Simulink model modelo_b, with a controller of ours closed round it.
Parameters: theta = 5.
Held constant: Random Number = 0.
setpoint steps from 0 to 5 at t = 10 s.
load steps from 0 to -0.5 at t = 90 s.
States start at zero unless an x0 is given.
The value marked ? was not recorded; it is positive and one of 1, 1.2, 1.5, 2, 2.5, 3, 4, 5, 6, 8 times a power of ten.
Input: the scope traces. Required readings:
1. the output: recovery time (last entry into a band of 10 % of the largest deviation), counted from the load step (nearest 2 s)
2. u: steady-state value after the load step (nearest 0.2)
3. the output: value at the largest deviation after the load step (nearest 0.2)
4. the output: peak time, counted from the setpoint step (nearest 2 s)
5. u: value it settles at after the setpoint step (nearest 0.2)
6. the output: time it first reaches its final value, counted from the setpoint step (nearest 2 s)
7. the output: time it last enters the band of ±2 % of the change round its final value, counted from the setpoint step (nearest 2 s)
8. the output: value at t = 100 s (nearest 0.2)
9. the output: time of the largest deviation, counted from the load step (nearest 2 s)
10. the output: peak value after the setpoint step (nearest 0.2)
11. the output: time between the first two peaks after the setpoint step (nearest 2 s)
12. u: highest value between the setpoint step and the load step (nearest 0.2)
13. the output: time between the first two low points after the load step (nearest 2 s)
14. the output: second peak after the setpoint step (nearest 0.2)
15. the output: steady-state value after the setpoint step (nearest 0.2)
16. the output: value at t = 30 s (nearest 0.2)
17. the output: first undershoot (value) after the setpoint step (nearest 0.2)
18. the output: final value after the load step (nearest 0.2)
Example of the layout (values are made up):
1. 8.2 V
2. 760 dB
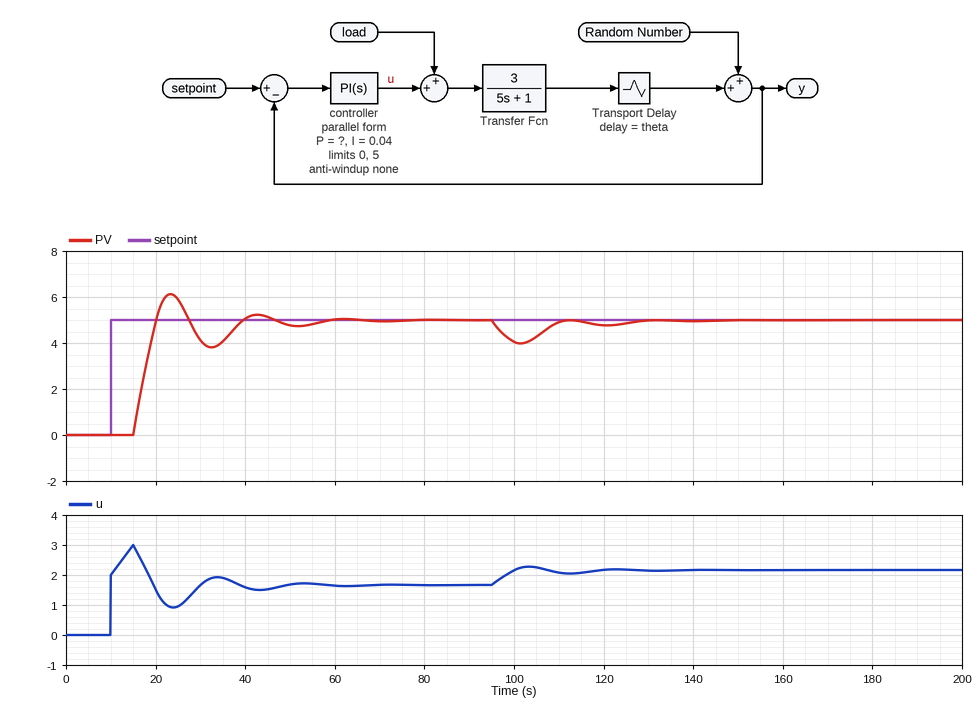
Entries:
1. 36 s
2. 2.2
3. 4.0
4. 14 s
5. 1.6
6. 10 s
7. 46 s
8. 4.0
9. 12 s
10. 6.2
11. 20 s
12. 3.0
13. 20 s
14. 5.2
15. 5.0
16. 4.2
17. 3.8
18. 5.0
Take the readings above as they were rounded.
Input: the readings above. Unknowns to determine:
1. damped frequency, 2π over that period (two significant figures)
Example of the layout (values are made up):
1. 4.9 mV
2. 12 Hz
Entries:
1. 0.31 rad/s
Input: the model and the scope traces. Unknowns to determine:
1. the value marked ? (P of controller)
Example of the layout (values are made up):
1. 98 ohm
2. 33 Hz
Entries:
1. 0.4
